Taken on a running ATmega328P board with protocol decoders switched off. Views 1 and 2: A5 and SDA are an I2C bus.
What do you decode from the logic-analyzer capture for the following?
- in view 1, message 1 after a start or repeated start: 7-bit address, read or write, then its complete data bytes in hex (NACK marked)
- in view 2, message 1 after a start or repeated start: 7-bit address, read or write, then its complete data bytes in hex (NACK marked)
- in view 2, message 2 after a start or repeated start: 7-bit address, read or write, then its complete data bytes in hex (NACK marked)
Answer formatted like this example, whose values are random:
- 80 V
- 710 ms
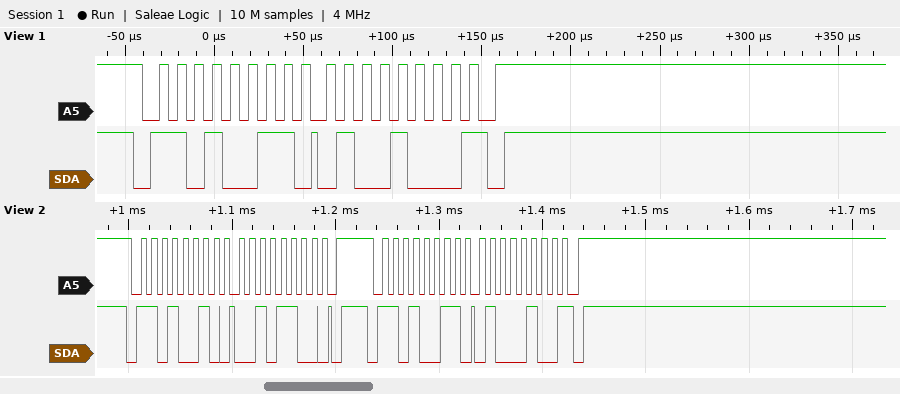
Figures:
- 0x69 read: 48 NACK
- 0x69 write: 2C
- 0x69 read: 44 NACK
